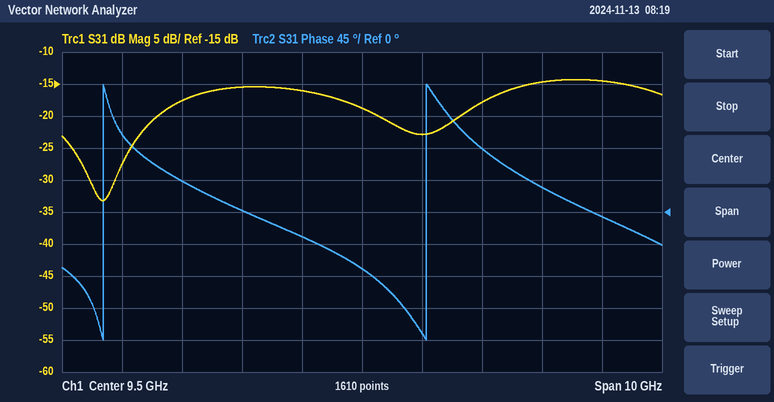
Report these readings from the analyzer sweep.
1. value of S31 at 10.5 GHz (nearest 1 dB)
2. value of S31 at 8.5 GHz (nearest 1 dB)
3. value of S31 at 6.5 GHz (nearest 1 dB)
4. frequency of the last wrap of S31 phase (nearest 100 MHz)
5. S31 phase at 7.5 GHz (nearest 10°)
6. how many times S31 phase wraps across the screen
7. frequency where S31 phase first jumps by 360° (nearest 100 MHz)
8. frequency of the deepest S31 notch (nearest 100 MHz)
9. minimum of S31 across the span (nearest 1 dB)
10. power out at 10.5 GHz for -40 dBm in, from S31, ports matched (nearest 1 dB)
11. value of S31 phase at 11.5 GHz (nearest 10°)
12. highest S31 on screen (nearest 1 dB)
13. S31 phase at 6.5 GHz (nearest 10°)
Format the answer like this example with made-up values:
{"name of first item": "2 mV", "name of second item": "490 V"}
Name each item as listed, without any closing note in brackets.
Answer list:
{"value of S31 at 10.5 GHz": "-23 dB", "value of S31 at 8.5 GHz": "-16 dB", "value of S31 at 6.5 GHz": "-18 dB", "frequency of the last wrap of S31 phase": "10.6 GHz", "S31 phase at 7.5 GHz": "0°", "how many times S31 phase wraps across the screen": "2", "frequency where S31 phase first jumps by 360°": "5.2 GHz", "frequency of the deepest S31 notch": "5.2 GHz", "minimum of S31 across the span": "-33 dB", "power out at 10.5 GHz for -40 dBm in, from S31, ports matched": "-63 dBm", "value of S31 phase at 11.5 GHz": "90°", "highest S31 on screen": "-14 dB", "S31 phase at 6.5 GHz": "40°"}
